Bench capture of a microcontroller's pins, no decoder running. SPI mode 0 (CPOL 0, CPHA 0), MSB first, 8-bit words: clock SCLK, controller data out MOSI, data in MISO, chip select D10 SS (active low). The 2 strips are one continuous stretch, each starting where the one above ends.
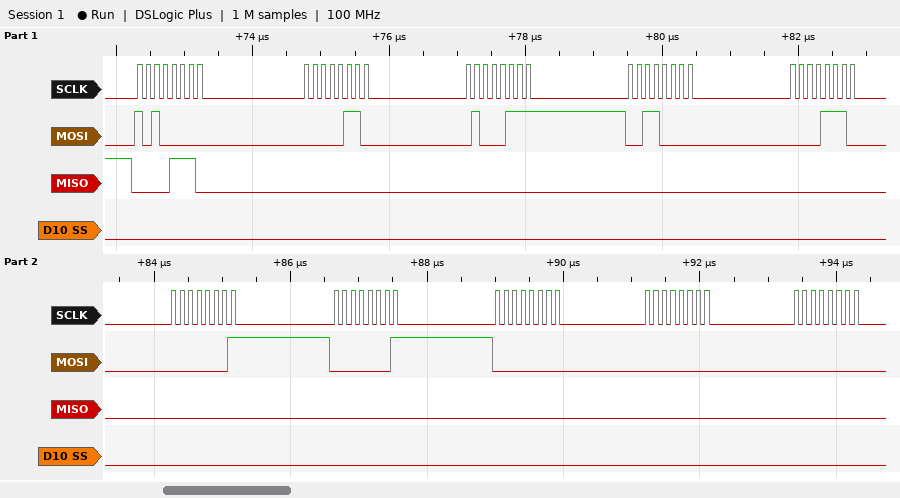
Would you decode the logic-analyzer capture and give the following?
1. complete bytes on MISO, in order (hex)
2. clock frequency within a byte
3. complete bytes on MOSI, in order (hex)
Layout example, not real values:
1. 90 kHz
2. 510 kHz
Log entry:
1. 0E 00 00 00 00 00 00 00 00 00
2. 8 MHz
3. A0 06 47 30 0E 01 01 00 00 00
